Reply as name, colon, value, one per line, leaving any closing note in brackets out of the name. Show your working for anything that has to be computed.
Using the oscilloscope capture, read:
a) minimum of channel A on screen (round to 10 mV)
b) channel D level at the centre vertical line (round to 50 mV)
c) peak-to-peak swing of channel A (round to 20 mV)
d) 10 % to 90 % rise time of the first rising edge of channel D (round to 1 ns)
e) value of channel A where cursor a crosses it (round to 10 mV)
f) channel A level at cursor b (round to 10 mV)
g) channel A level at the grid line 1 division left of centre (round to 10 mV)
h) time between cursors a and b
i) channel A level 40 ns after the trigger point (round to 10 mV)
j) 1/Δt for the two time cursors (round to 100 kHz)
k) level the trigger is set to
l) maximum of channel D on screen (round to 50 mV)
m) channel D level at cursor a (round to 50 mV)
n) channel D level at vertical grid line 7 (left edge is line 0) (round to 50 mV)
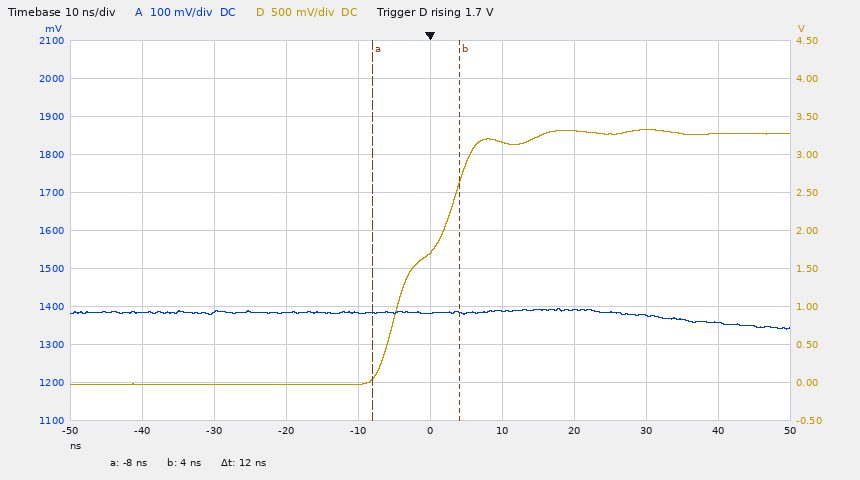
minimum of channel A on screen: 1.34 V
channel D level at the centre vertical line: 1.70 V
peak-to-peak swing of channel A: 60 mV
10 % to 90 % rise time of the first rising edge of channel D: 12 ns
value of channel A where cursor a crosses it: 1.38 V
channel A level at cursor b: 1.38 V
channel A level at the grid line 1 division left of centre: 1.38 V
time between cursors a and b: 12 ns
channel A level 40 ns after the trigger point: 1.36 V
1/Δt for the two time cursors: 1 / 12 ns ≈ 83.3 MHz
level the trigger is set to: 1.7 V
maximum of channel D on screen: 3.35 V
channel D level at cursor a: 50 mV
channel D level at vertical grid line 7 (left edge is line 0): 3.30 V
